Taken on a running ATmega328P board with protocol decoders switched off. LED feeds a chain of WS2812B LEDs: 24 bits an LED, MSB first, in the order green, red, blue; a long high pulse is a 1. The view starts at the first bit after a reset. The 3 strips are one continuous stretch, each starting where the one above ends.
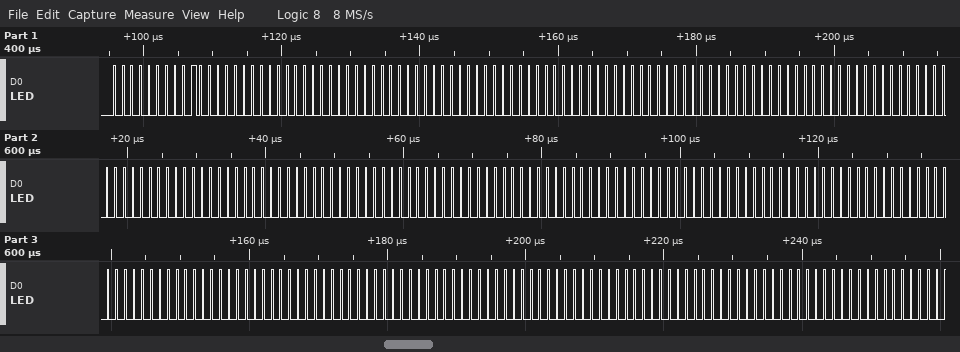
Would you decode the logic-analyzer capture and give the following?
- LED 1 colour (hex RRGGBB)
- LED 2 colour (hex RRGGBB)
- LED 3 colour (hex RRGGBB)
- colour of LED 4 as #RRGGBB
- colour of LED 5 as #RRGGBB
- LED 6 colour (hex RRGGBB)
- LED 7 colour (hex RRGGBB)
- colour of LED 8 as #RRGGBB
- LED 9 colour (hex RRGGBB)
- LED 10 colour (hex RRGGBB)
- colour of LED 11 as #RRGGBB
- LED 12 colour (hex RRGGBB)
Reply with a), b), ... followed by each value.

a) #400000
b) #000000
c) #000000
d) #000000
e) #000000
f) #000000
g) #000000
h) #000000
i) #000000
j) #000000
k) #000000
l) #000000
